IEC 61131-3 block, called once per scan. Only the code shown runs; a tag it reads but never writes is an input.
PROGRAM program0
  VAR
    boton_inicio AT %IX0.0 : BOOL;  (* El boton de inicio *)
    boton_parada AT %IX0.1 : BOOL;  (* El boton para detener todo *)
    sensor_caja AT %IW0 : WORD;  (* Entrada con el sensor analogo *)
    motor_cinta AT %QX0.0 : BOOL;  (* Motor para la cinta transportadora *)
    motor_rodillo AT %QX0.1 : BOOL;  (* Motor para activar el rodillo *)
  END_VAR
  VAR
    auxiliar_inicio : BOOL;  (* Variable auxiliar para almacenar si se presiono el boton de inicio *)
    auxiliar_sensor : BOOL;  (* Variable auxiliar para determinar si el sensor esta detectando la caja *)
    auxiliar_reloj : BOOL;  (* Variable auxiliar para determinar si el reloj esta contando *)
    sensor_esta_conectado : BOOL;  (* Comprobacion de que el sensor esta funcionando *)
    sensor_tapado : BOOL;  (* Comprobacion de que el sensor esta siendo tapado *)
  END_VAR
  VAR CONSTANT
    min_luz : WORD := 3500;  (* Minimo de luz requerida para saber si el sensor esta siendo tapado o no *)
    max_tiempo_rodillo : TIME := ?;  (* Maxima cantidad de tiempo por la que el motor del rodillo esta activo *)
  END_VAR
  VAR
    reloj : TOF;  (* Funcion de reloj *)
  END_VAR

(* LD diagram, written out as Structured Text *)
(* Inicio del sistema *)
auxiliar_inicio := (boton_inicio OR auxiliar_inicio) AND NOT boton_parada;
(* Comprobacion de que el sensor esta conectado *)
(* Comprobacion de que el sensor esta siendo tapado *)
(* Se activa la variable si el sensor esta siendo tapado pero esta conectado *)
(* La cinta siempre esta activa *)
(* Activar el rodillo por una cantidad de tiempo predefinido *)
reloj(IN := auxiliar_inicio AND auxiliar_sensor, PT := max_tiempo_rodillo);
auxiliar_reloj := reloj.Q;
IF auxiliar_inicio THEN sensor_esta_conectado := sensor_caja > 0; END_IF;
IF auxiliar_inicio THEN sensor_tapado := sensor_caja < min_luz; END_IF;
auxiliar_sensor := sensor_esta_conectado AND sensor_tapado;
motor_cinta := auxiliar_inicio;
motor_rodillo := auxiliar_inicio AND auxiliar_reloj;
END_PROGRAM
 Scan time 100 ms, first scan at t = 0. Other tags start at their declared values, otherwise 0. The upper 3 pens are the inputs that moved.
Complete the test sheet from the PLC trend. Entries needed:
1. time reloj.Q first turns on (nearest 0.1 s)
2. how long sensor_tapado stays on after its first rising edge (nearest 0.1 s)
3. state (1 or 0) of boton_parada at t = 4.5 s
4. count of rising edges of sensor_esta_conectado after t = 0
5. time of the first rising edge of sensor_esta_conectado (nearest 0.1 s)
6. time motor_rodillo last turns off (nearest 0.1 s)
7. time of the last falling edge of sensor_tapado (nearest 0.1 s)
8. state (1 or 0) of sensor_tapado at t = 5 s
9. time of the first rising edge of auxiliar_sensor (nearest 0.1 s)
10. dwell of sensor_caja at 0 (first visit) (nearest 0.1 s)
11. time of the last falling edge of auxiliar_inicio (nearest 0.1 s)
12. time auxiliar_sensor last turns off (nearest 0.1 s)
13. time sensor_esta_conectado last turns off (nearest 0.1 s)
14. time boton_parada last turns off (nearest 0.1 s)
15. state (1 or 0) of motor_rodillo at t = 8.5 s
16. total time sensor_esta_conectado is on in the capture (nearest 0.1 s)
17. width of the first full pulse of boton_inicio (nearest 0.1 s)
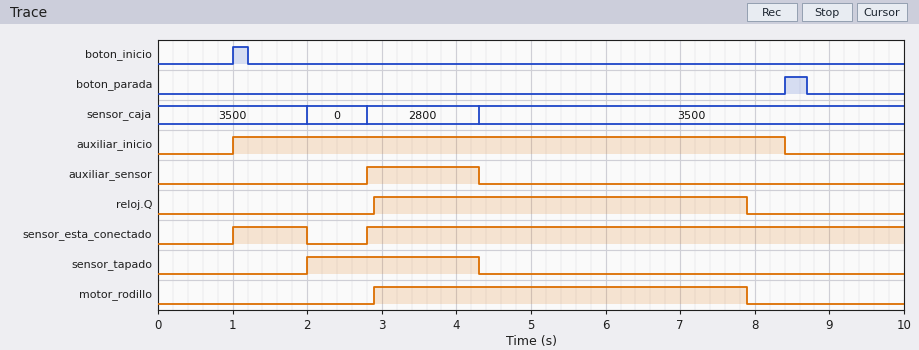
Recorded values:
2.9 s
2.3 s
0
2
1.0 s
7.9 s
4.3 s
0
2.8 s
0.8 s
8.4 s
4.3 s
2.0 s
8.7 s
0
8.2 s
0.2 s
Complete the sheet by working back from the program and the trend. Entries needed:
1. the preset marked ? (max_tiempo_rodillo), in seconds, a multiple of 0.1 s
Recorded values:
3.5 s
